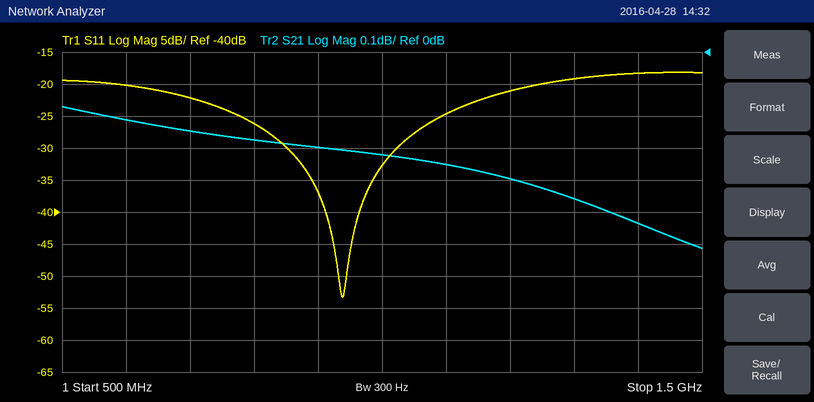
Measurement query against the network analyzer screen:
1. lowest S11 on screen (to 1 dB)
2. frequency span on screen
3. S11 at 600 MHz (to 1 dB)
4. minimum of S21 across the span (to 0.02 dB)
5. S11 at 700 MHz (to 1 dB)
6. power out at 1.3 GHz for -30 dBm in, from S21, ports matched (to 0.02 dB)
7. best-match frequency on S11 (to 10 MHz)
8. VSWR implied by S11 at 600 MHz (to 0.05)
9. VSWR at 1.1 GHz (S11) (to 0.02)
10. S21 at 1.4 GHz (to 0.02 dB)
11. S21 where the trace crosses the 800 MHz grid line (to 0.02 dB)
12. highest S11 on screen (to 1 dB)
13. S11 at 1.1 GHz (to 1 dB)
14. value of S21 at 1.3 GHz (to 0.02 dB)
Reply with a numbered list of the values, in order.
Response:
1. -53 dB
2. 1 GHz
3. -20 dB
4. -0.62 dB
5. -22 dB
6. -30.46 dBm
7. 940 MHz
8. 1.20
9. 1.12
10. -0.54 dB
11. -0.28 dB
12. -18 dB
13. -25 dB
14. -0.46 dB
